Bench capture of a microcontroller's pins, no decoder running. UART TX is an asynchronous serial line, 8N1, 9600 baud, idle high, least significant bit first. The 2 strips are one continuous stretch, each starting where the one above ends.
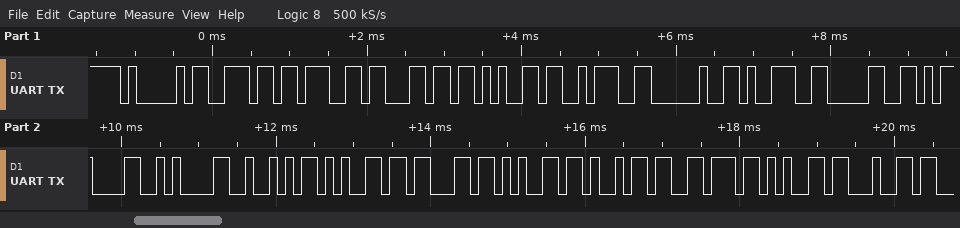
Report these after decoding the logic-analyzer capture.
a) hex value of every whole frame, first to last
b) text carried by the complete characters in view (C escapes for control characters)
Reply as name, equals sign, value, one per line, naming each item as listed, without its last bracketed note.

hex value of every whole frame, first to last = 41 6E 67 6C 65 3A 20 39 30 0D 0A 52 65 63 65 69 76 65 64
text carried by the complete characters in view = "Angle: 90\r\nReceived"
